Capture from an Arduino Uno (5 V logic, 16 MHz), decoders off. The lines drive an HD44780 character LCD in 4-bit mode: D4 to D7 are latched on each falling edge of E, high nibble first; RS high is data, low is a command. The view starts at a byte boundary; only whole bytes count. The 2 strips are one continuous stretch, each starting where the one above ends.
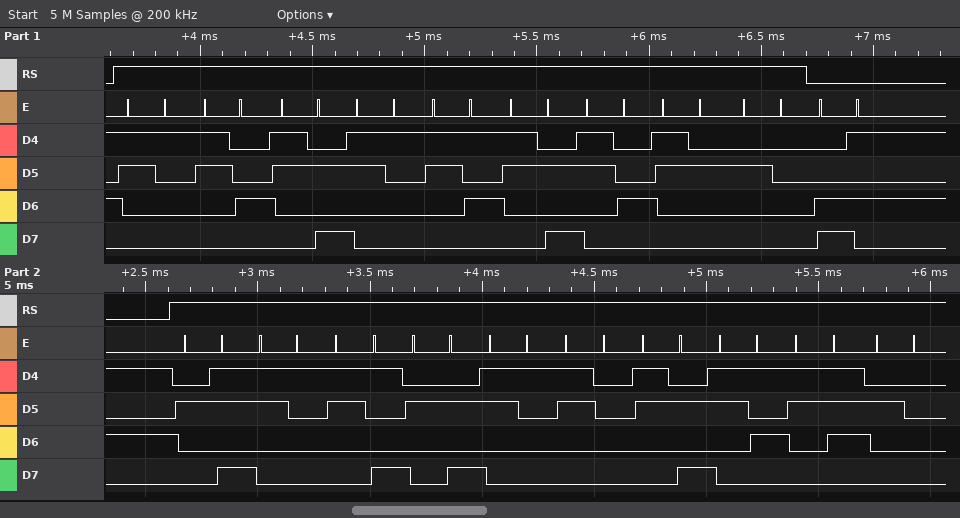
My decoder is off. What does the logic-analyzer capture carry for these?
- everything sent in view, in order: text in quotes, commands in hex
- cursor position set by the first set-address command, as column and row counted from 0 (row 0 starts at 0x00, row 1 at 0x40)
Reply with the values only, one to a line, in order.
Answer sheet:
"14:15:42 " 0xC5 "+19*10:57 "
column 5, row 1
